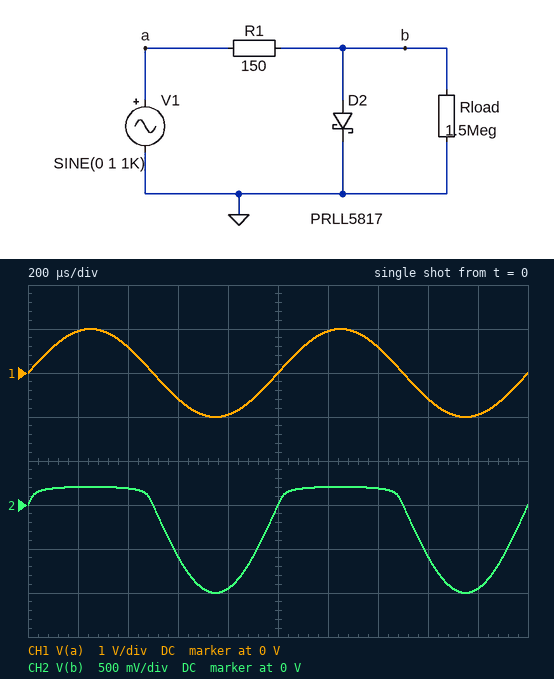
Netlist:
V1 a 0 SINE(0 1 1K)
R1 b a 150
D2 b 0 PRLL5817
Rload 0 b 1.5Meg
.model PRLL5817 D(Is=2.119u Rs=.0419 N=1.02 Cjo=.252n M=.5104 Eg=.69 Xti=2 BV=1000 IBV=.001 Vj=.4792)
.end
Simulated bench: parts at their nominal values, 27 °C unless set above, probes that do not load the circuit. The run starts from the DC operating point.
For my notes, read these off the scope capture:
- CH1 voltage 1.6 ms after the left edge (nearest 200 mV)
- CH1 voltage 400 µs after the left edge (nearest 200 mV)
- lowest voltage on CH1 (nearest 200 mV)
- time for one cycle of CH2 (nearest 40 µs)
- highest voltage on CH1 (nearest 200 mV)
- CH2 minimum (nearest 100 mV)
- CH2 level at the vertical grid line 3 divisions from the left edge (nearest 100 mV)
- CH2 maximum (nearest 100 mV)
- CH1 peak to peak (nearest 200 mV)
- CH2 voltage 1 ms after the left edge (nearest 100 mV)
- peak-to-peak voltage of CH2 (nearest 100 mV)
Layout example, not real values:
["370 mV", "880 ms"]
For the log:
["-600 mV", "600 mV", "-1.0 V", "1.00 ms", "1.0 V", "-1.0 V", "-600 mV", "200 mV", "2.0 V", "0 V", "1.2 V"]
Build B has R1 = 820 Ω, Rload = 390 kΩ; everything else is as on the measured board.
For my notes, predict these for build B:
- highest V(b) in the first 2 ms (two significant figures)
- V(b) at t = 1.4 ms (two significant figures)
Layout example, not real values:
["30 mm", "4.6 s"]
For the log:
["160 mV", "150 mV"]
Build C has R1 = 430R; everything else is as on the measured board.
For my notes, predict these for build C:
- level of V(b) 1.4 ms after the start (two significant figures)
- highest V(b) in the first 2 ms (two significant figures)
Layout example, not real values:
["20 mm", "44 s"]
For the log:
["160 mV", "180 mV"]
